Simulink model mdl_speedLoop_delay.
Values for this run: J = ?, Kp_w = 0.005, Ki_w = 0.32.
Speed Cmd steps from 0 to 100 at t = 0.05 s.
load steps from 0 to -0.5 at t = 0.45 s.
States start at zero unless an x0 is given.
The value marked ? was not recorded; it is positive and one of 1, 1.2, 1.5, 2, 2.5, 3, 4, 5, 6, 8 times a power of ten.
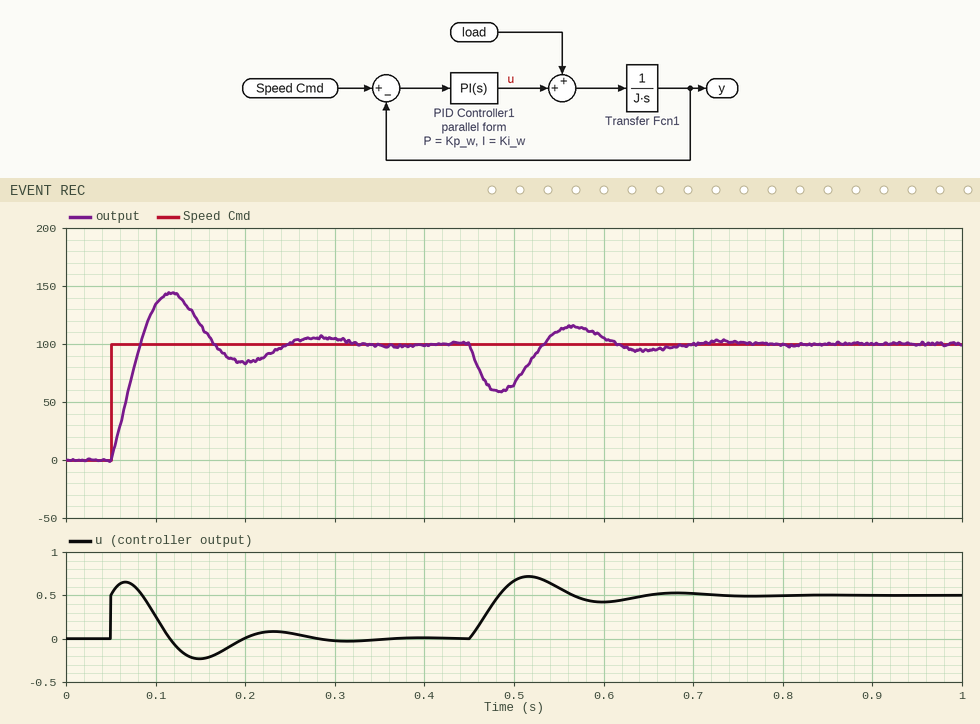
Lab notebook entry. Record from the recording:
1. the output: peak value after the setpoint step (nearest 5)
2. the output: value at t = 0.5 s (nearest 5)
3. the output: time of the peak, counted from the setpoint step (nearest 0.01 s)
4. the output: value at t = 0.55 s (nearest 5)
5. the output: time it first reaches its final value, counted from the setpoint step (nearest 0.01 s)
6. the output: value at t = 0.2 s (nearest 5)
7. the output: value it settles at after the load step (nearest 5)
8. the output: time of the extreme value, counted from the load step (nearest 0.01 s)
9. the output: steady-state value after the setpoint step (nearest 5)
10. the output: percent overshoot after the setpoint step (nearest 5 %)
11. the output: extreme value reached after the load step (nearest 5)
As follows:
145
65
0.07 s
110
0.03 s
85
100
0.03 s
100
45 %
60
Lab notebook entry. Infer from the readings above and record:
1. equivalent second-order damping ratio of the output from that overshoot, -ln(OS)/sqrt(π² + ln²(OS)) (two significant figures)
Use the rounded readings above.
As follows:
0.25
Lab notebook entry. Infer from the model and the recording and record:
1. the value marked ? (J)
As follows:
0.0002
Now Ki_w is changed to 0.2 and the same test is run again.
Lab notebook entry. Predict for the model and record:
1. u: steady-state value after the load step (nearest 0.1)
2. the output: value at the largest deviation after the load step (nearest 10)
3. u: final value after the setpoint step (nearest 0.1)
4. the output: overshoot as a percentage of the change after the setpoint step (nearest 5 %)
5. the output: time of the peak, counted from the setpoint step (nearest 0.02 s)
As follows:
0.5
50
0.0
35 %
0.08 s
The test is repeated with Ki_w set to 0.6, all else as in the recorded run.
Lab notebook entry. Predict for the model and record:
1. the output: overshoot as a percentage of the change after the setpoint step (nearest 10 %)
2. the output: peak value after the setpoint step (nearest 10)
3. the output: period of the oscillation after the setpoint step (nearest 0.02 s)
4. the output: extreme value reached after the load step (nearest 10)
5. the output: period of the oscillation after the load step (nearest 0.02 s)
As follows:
50 %
150
0.12 s
70
0.12 s
